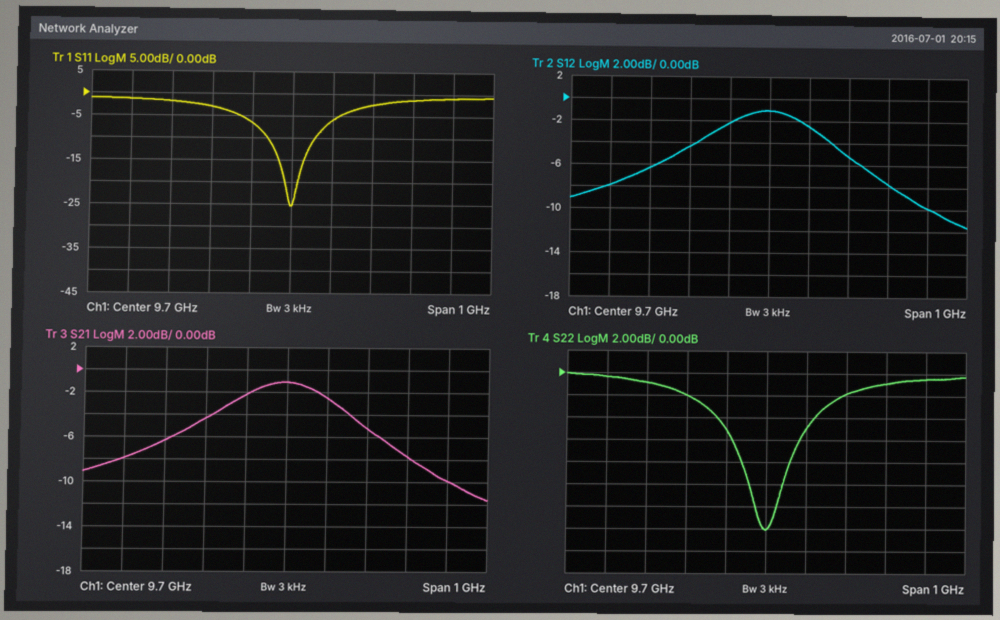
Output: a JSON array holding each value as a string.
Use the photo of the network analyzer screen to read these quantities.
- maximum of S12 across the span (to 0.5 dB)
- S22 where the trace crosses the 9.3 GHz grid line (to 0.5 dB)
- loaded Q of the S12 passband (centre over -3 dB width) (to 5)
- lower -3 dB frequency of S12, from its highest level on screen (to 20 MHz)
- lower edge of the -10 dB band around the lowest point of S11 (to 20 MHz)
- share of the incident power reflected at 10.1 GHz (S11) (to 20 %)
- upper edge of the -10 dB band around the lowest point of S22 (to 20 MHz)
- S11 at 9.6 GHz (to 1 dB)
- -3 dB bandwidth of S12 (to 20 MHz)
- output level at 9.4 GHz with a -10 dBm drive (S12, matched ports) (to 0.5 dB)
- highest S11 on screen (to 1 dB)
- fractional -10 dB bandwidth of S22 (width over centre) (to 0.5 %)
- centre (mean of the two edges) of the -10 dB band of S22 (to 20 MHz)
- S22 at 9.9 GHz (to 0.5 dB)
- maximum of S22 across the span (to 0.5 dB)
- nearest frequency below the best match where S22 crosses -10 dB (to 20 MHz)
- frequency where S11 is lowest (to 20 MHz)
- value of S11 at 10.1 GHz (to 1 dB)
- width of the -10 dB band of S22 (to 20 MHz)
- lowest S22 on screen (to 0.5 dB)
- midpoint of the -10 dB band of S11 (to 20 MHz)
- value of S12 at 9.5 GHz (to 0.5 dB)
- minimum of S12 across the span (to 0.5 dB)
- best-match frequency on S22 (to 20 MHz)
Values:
["-1.0 dB", "-0.5 dB", "30", "9.52 GHz", "9.64 GHz", "80 %", "9.74 GHz", "-7 dB", "340 MHz", "-16.5 dBm", "-1 dB", "1.0 %", "9.70 GHz", "-2.0 dB", "0.0 dB", "9.66 GHz", "9.70 GHz", "-1 dB", "80 MHz", "-14.0 dB", "9.70 GHz", "-4.5 dB", "-11.5 dB", "9.70 GHz"]
